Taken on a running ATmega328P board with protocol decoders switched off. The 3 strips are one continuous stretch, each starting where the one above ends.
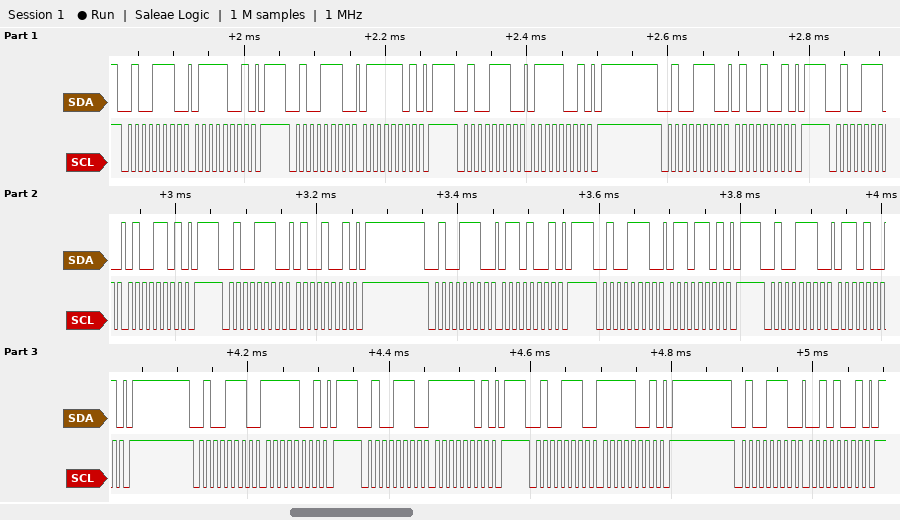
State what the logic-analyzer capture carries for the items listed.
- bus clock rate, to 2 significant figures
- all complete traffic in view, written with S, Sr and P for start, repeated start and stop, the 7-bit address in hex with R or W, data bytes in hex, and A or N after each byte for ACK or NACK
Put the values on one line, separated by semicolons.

100 kHz; S 27W A 79 A P S 27W A 7D A P S 27W A 79 A P S 27W A 49 A P S 27W A 4D A P S 27W A 49 A P S 27W A 69 A P S 27W A 6D A P S 27W A 69 A P S 27W A F9 A P S 27W A FD A P S 27W A F9 A P S 27W A 29 A P
